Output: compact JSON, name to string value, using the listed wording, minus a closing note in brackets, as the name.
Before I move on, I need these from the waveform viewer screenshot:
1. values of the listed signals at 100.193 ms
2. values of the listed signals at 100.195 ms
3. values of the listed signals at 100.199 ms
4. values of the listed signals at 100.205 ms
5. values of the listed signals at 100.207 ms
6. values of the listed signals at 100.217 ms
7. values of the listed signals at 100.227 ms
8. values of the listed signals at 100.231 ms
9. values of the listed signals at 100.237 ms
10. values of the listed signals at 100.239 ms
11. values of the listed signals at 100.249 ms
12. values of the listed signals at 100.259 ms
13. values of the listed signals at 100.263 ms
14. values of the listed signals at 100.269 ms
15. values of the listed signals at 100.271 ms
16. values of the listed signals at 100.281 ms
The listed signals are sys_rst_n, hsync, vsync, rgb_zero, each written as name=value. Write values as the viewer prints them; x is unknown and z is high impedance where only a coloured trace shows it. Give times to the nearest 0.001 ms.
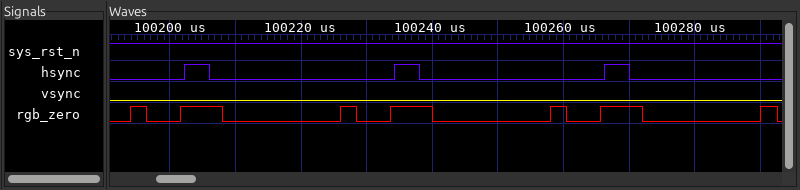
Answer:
{"values of the listed signals at 100.193 ms": "sys_rst_n=1, hsync=0, vsync=0, rgb_zero=0", "values of the listed signals at 100.195 ms": "sys_rst_n=1, hsync=0, vsync=0, rgb_zero=1", "values of the listed signals at 100.199 ms": "sys_rst_n=1, hsync=0, vsync=0, rgb_zero=0", "values of the listed signals at 100.205 ms": "sys_rst_n=1, hsync=1, vsync=0, rgb_zero=1", "values of the listed signals at 100.207 ms": "sys_rst_n=1, hsync=0, vsync=0, rgb_zero=1", "values of the listed signals at 100.217 ms": "sys_rst_n=1, hsync=0, vsync=0, rgb_zero=0", "values of the listed signals at 100.227 ms": "sys_rst_n=1, hsync=0, vsync=0, rgb_zero=1", "values of the listed signals at 100.231 ms": "sys_rst_n=1, hsync=0, vsync=0, rgb_zero=0", "values of the listed signals at 100.237 ms": "sys_rst_n=1, hsync=1, vsync=0, rgb_zero=1", "values of the listed signals at 100.239 ms": "sys_rst_n=1, hsync=0, vsync=0, rgb_zero=1", "values of the listed signals at 100.249 ms": "sys_rst_n=1, hsync=0, vsync=0, rgb_zero=0", "values of the listed signals at 100.259 ms": "sys_rst_n=1, hsync=0, vsync=0, rgb_zero=1", "values of the listed signals at 100.263 ms": "sys_rst_n=1, hsync=0, vsync=0, rgb_zero=0", "values of the listed signals at 100.269 ms": "sys_rst_n=1, hsync=1, vsync=0, rgb_zero=1", "values of the listed signals at 100.271 ms": "sys_rst_n=1, hsync=0, vsync=0, rgb_zero=1", "values of the listed signals at 100.281 ms": "sys_rst_n=1, hsync=0, vsync=0, rgb_zero=0"}
